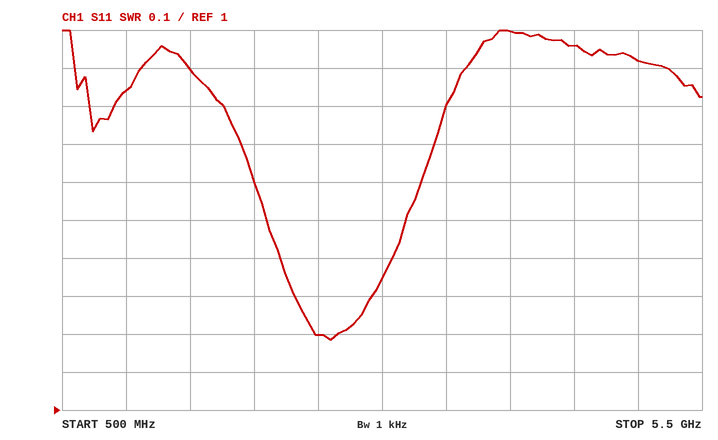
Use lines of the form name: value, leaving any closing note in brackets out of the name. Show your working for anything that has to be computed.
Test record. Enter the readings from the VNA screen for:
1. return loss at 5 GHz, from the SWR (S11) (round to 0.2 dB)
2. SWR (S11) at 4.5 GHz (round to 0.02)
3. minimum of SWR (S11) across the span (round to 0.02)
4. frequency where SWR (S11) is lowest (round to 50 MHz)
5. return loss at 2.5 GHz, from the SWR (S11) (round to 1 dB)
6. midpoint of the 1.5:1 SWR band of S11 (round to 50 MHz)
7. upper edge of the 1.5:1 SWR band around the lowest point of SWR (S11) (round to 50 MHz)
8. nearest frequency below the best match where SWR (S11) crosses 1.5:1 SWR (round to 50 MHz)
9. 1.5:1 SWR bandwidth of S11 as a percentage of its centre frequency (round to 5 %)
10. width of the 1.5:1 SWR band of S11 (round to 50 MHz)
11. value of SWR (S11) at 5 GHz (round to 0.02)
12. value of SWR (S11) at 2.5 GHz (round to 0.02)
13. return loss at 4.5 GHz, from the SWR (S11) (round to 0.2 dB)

return loss at 5 GHz, from the SWR (S11): −20 log10((1.92 − 1)/(1.92 + 1)) ≈ 10.0 dB
SWR (S11) at 4.5 GHz: 1.96
minimum of SWR (S11) across the span: 1.18
frequency where SWR (S11) is lowest: 2.60 GHz
return loss at 2.5 GHz, from the SWR (S11): −20 log10((1.2 − 1)/(1.2 + 1)) ≈ 21 dB
midpoint of the 1.5:1 SWR band of S11: 2.65 GHz
upper edge of the 1.5:1 SWR band around the lowest point of SWR (S11): 3.20 GHz
nearest frequency below the best match where SWR (S11) crosses 1.5:1 SWR: 2.10 GHz
1.5:1 SWR bandwidth of S11 as a percentage of its centre frequency: 1.1 GHz / 2.65 GHz ≈ 41.5 %, so 40 % to the nearest 5 %
width of the 1.5:1 SWR band of S11: 3.20 GHz − 2.10 GHz = 1.10 GHz
value of SWR (S11) at 5 GHz: 1.92
value of SWR (S11) at 2.5 GHz: 1.20
return loss at 4.5 GHz, from the SWR (S11): −20 log10((1.96 − 1)/(1.96 + 1)) ≈ 9.8 dB
